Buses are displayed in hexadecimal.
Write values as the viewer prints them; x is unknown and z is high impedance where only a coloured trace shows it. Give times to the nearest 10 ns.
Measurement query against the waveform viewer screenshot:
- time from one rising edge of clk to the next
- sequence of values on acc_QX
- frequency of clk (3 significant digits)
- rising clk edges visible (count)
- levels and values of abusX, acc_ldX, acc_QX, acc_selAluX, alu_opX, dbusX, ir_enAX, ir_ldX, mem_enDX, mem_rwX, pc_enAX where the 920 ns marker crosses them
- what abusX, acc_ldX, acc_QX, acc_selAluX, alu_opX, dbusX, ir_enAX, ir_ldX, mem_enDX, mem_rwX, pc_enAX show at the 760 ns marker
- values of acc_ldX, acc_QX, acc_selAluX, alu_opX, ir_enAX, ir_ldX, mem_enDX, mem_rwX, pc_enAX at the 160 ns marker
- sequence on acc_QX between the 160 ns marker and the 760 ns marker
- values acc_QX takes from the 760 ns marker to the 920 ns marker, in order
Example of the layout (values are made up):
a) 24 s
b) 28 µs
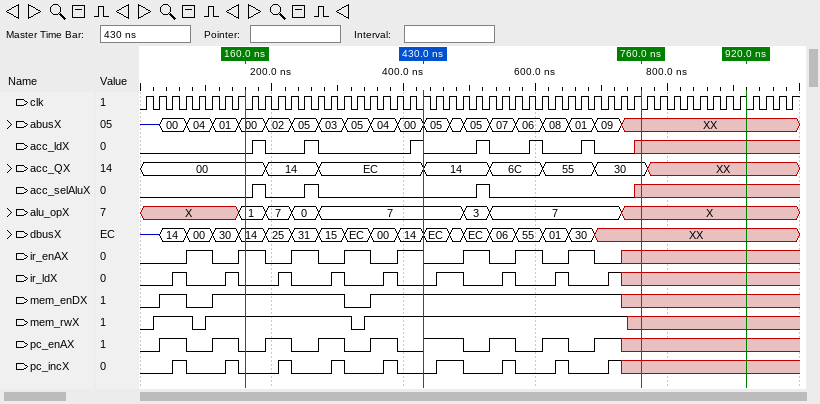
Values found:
a) 20 ns
b) 00, 14, EC, 14, 6C, 55, 30, XX
c) 50.0 MHz
d) 50
e) abusX=XX, acc_ldX=x, acc_QX=XX, acc_selAluX=x, alu_opX=X, dbusX=XX, ir_enAX=x, ir_ldX=x, mem_enDX=x, mem_rwX=x, pc_enAX=x
f) abusX=XX, acc_ldX=x, acc_QX=30, acc_selAluX=x, alu_opX=X, dbusX=XX, ir_enAX=x, ir_ldX=x, mem_enDX=x, mem_rwX=x, pc_enAX=x
g) acc_ldX=0, acc_QX=00, acc_selAluX=0, alu_opX=1, ir_enAX=1, ir_ldX=0, mem_enDX=1, mem_rwX=1, pc_enAX=0
h) 00, 14, EC, 14, 6C, 55, 30
i) 30, XX
